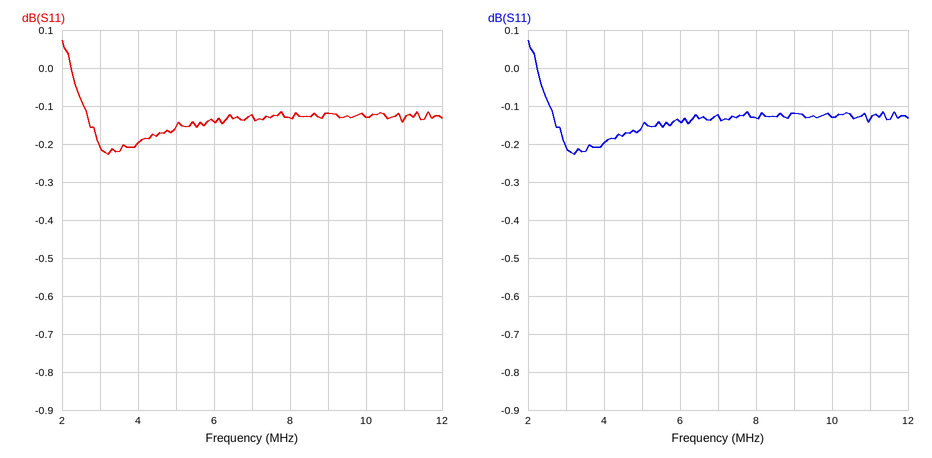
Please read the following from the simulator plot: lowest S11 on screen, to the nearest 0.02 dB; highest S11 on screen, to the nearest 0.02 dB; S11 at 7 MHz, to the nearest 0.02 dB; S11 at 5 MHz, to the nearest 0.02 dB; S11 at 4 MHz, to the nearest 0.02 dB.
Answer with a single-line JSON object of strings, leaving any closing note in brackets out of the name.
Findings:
{"lowest S11 on screen, to the nearest 0.02 dB": "-0.22 dB", "highest S11 on screen, to the nearest 0.02 dB": "0.08 dB", "S11 at 7 MHz, to the nearest 0.02 dB": "-0.12 dB", "S11 at 5 MHz, to the nearest 0.02 dB": "-0.16 dB", "S11 at 4 MHz, to the nearest 0.02 dB": "-0.20 dB"}
